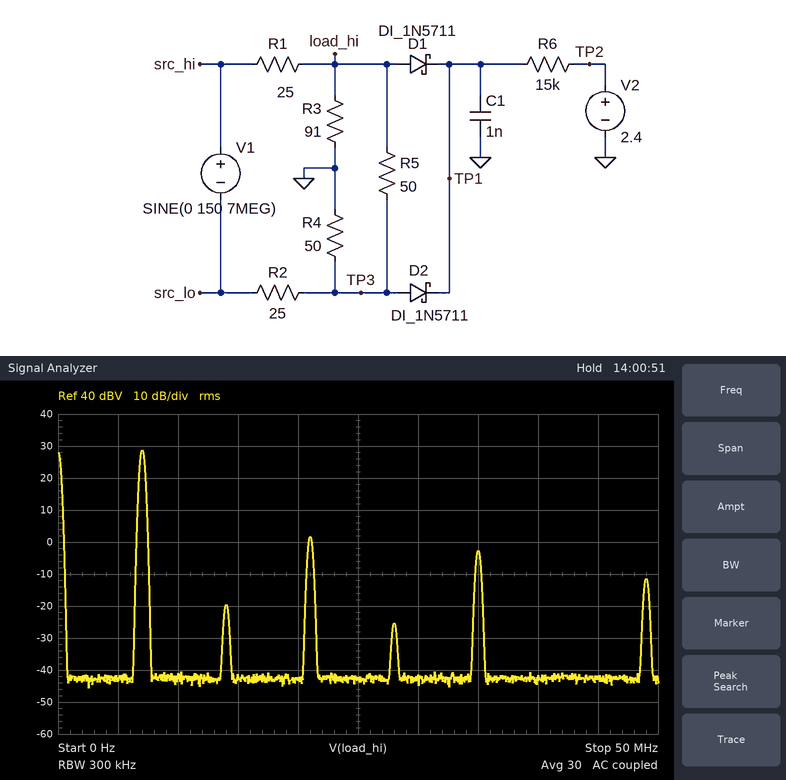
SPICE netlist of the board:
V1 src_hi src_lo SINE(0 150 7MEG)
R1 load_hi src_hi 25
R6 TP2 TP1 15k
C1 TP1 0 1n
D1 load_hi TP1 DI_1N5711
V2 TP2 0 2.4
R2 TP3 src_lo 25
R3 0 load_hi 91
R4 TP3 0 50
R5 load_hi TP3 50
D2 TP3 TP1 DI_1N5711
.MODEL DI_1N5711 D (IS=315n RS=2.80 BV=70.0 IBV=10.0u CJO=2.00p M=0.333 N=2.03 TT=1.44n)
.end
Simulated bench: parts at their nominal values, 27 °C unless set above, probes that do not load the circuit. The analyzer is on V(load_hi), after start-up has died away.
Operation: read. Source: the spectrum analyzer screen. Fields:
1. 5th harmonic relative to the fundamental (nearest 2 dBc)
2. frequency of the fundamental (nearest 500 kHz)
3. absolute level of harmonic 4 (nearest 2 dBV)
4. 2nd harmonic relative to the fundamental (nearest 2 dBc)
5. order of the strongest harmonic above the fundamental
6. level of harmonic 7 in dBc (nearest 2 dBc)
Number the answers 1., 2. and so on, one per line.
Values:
1. -32 dBc
2. 7.0 MHz
3. -26 dBV
4. -48 dBc
5. 3
6. -40 dBc
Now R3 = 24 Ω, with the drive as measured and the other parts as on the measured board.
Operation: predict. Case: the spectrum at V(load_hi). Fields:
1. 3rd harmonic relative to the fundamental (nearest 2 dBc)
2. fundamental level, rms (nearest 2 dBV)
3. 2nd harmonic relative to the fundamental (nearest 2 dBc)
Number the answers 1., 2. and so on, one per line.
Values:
1. -38 dBc
2. 22 dBV
3. -52 dBc
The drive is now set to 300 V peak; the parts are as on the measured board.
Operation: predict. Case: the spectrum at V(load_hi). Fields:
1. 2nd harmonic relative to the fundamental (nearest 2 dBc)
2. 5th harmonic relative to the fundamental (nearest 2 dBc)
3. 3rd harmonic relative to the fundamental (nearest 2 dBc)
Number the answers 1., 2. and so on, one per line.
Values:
1. -58 dBc
2. -24 dBc
3. -16 dBc
